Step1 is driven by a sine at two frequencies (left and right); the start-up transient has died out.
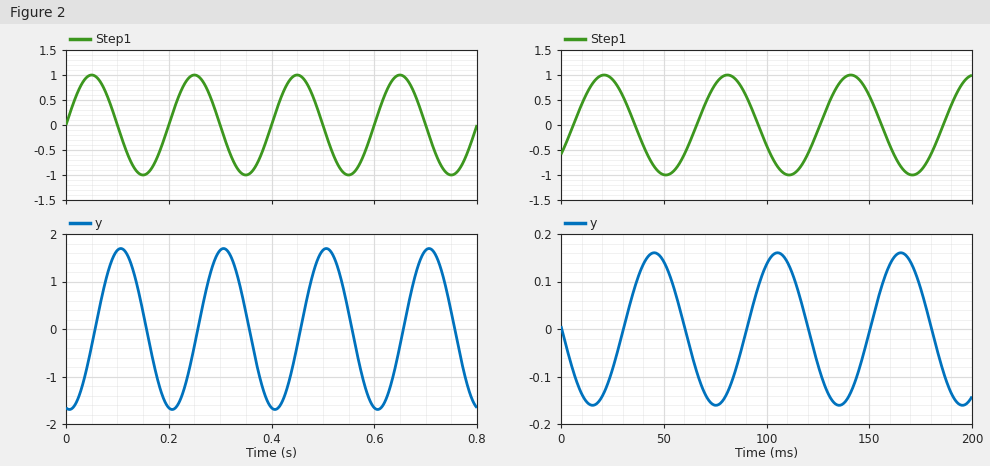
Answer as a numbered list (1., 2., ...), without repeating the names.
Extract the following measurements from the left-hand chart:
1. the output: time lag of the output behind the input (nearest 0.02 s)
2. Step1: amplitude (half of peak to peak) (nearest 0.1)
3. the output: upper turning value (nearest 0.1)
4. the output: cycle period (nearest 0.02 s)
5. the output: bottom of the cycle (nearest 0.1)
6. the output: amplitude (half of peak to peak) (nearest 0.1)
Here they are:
1. 0.06 s
2. 1.0
3. 1.7
4. 0.20 s
5. -1.7
6. 1.7
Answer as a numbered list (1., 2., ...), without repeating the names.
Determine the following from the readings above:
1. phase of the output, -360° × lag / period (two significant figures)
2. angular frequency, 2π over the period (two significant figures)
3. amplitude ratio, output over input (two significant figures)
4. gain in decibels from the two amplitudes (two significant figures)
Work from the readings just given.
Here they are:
1. -110°
2. 31 rad/s
3. 1.7
4. 4.6 dB
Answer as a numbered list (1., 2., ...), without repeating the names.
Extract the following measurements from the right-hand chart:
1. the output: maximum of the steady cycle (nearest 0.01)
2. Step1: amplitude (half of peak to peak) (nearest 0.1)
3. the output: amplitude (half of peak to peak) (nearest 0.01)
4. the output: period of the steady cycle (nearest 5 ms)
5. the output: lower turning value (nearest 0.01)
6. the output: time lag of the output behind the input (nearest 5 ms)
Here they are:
1. 0.16
2. 1.0
3. 0.16
4. 60 ms
5. -0.16
6. 25 ms
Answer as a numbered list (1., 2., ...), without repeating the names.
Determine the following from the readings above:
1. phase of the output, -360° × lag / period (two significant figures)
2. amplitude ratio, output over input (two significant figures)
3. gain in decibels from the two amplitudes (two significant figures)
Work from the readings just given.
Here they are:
1. -150°
2. 0.16
3. -16 dB
